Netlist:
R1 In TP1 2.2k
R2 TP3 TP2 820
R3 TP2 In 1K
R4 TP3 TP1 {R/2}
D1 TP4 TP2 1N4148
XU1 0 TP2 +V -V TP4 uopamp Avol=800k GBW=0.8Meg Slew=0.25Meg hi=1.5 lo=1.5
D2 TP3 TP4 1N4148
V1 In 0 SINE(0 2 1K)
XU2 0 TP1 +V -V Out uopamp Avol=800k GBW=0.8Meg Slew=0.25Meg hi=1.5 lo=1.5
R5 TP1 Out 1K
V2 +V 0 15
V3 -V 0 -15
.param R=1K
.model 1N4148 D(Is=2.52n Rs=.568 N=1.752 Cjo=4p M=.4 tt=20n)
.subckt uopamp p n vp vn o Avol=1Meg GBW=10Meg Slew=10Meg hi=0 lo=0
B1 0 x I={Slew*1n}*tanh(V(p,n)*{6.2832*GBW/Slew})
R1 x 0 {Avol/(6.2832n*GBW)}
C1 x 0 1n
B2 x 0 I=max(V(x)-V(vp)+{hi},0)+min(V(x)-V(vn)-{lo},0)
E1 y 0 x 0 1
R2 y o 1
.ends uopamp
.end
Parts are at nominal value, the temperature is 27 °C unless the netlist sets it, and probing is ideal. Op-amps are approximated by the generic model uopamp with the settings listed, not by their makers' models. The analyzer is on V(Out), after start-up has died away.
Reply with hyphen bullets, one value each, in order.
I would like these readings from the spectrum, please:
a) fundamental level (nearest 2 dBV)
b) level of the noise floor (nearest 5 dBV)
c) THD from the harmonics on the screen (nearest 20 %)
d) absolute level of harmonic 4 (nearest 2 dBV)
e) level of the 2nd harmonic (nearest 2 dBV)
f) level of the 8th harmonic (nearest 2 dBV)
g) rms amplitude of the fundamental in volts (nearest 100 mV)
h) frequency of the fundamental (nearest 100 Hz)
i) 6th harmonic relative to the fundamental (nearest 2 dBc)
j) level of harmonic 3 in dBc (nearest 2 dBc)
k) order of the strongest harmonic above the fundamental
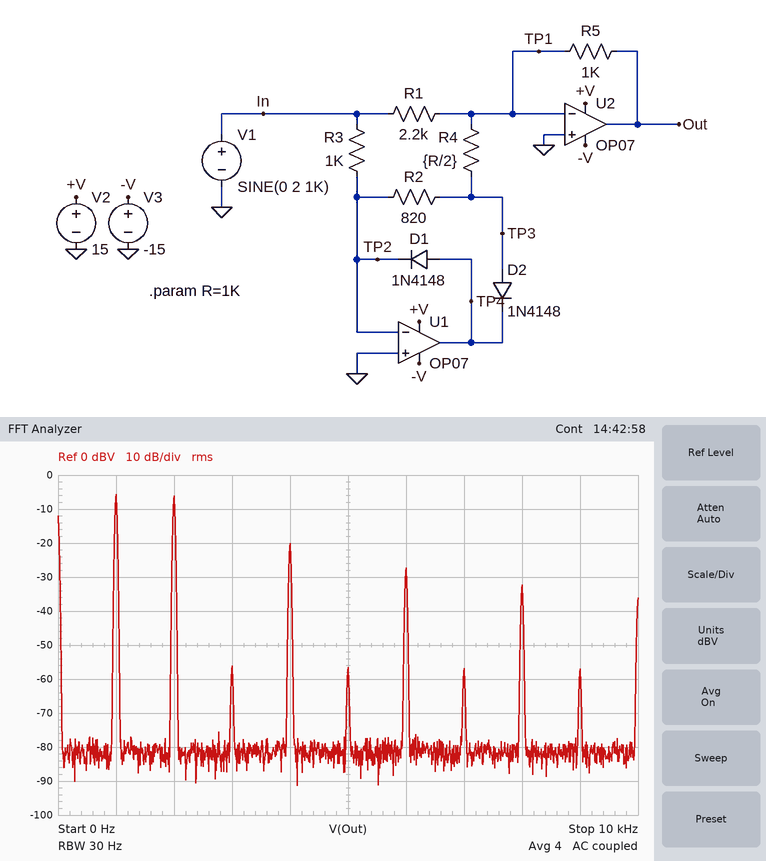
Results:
- -6 dBV
- -80 dBV
- 100 %
- -20 dBV
- -6 dBV
- -32 dBV
- 500 mV
- 1.0 kHz
- -22 dBc
- -50 dBc
- 2
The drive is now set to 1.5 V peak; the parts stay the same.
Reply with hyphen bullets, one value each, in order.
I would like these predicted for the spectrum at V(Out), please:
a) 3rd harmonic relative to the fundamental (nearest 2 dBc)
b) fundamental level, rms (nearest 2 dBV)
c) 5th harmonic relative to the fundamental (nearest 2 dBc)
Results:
- -48 dBc
- -8 dBV
- -48 dBc
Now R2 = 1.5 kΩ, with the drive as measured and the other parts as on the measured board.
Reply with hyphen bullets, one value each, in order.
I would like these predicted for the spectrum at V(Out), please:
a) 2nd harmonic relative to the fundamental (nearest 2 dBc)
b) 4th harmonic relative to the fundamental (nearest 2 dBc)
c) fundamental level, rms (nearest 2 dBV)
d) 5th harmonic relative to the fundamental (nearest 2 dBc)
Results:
- -4 dBc
- -18 dBc
- 4 dBV
- -58 dBc
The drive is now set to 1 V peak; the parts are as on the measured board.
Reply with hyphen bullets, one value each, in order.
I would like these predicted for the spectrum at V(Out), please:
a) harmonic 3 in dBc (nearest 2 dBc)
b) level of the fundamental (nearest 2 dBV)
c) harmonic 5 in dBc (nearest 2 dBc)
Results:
- -46 dBc
- -12 dBV
- -46 dBc
